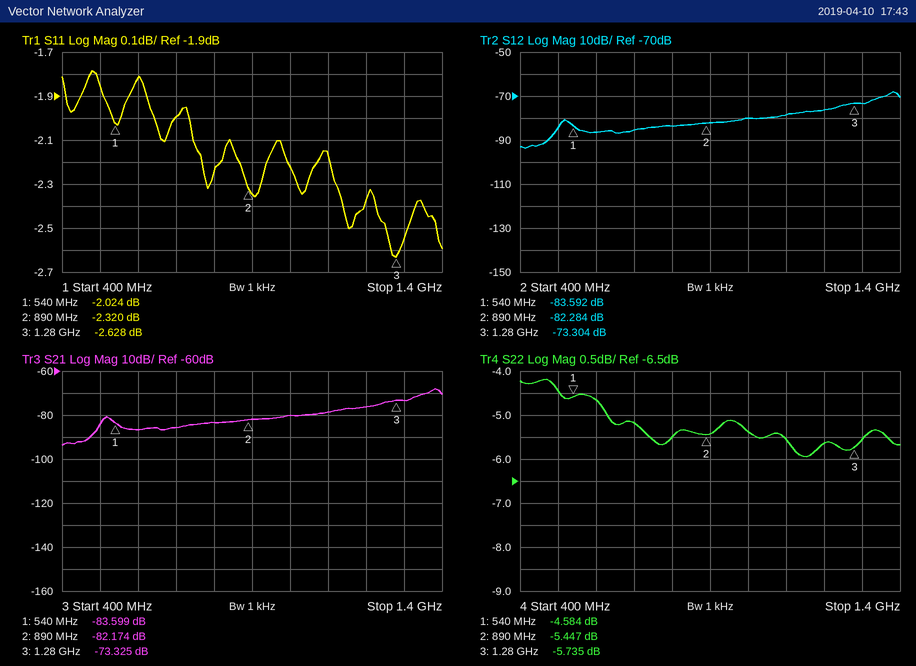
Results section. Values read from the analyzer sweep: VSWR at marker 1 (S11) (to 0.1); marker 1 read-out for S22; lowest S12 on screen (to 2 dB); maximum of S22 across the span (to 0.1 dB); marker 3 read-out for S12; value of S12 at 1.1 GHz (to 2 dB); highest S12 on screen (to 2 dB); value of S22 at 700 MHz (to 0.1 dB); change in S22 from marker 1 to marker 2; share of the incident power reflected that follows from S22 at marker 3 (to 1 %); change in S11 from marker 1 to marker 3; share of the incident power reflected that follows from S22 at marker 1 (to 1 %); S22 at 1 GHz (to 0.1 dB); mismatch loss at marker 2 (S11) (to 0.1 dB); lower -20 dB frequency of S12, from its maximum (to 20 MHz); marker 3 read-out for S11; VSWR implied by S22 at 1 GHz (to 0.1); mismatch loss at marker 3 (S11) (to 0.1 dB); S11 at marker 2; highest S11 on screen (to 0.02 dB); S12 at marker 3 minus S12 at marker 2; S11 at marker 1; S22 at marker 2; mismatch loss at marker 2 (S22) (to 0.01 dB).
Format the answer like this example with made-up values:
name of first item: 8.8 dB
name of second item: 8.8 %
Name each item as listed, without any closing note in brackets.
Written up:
VSWR at marker 1 (S11): 8.6
marker 1 read-out for S22: -4.584 dB
lowest S12 on screen: -94 dB
maximum of S22 across the span: -4.2 dB
marker 3 read-out for S12: -73.304 dB
value of S12 at 1.1 GHz: -78 dB
highest S12 on screen: -68 dB
value of S22 at 700 MHz: -5.2 dB
change in S22 from marker 1 to marker 2: -0.863 dB
share of the incident power reflected that follows from S22 at marker 3: 27 %
change in S11 from marker 1 to marker 3: -0.604 dB
share of the incident power reflected that follows from S22 at marker 1: 35 %
S22 at 1 GHz: -5.4 dB
mismatch loss at marker 2 (S11): 3.8 dB
lower -20 dB frequency of S12, from its maximum: 480 MHz
marker 3 read-out for S11: -2.628 dB
VSWR implied by S22 at 1 GHz: 3.3
mismatch loss at marker 3 (S11): 3.4 dB
S11 at marker 2: -2.320 dB
highest S11 on screen: -1.78 dB
S12 at marker 3 minus S12 at marker 2: 8.980 dB
S11 at marker 1: -2.024 dB
S22 at marker 2: -5.447 dB
mismatch loss at marker 2 (S22): 1.46 dB
